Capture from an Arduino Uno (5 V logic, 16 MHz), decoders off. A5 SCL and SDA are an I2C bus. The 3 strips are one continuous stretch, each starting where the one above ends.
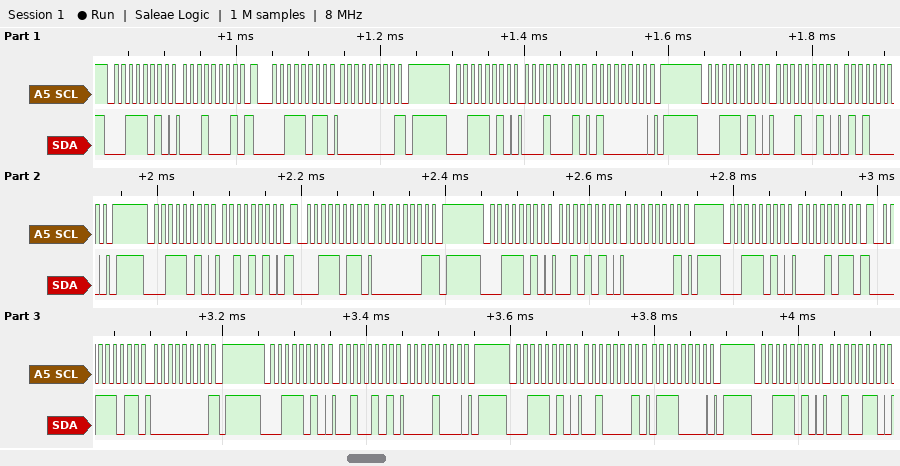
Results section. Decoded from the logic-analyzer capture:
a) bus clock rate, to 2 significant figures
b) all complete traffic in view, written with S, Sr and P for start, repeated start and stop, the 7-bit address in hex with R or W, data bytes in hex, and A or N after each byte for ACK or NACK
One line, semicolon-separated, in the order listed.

100 kHz; S 1DW A 11 A Sr 1DR A 00 N P S 1DW A 11 A 40 A P S 1DW A 12 A 50 A P S 1DW A 2A A Sr 1DR A 01 N P S 1DW A 2A A 01 A P S 1DW A 0B A Sr 1DR A 00 N P S 1DW A 25 A 08 A P S 1DW A 21 A 70 A P S 1DW A 26 A
